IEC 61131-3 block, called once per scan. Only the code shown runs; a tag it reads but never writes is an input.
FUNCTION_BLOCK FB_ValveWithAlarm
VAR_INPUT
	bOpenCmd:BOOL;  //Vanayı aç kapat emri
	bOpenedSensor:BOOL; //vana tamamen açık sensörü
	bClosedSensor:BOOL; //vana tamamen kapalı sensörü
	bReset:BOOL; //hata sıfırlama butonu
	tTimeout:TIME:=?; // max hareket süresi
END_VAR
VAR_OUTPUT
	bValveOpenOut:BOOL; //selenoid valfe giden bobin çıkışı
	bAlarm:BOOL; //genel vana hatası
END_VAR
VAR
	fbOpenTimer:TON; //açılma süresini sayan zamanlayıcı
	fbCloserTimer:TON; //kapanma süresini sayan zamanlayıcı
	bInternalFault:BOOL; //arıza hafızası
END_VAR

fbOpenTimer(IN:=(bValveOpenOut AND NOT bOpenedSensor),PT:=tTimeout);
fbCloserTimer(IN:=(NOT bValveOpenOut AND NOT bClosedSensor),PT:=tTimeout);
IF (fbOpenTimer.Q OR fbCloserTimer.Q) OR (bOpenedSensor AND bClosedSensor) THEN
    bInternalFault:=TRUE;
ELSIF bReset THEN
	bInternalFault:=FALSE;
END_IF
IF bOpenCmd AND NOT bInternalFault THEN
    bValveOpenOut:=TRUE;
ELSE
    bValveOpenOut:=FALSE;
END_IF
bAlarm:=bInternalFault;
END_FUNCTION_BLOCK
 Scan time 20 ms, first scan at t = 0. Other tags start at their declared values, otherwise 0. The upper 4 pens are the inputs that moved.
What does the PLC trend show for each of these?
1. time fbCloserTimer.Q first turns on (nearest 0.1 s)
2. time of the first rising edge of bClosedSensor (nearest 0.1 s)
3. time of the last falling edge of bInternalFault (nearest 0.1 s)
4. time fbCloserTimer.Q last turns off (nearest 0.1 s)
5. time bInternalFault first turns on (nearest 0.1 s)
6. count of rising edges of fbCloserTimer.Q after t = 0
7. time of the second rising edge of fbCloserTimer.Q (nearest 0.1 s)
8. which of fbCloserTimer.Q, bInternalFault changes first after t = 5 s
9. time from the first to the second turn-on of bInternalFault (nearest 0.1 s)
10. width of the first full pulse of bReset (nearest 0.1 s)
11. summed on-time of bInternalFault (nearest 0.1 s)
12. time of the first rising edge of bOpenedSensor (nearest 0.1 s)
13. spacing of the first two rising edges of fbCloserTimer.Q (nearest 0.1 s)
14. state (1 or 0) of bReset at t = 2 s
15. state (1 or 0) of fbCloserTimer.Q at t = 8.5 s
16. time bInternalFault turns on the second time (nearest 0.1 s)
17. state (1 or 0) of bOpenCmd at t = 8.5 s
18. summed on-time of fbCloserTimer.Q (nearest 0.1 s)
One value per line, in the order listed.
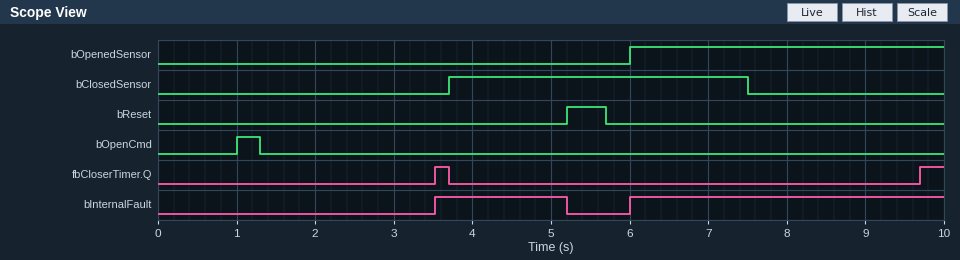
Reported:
3.5 s
3.7 s
5.2 s
3.7 s
3.5 s
2
9.7 s
bInternalFault
2.5 s
0.5 s
5.7 s
6.0 s
6.2 s
0
0
6.0 s
0
0.5 s
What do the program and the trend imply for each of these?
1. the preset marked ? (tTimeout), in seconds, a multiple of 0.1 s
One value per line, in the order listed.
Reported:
2.2 s
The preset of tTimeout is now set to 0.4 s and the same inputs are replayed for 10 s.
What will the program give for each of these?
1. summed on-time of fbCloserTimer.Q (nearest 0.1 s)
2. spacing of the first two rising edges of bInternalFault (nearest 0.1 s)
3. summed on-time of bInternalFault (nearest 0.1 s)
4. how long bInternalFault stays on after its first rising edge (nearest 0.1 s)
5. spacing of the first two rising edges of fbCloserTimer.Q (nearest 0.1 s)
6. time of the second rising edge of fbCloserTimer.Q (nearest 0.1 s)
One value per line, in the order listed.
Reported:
5.4 s
5.6 s
8.8 s
4.8 s
7.5 s
7.9 s
